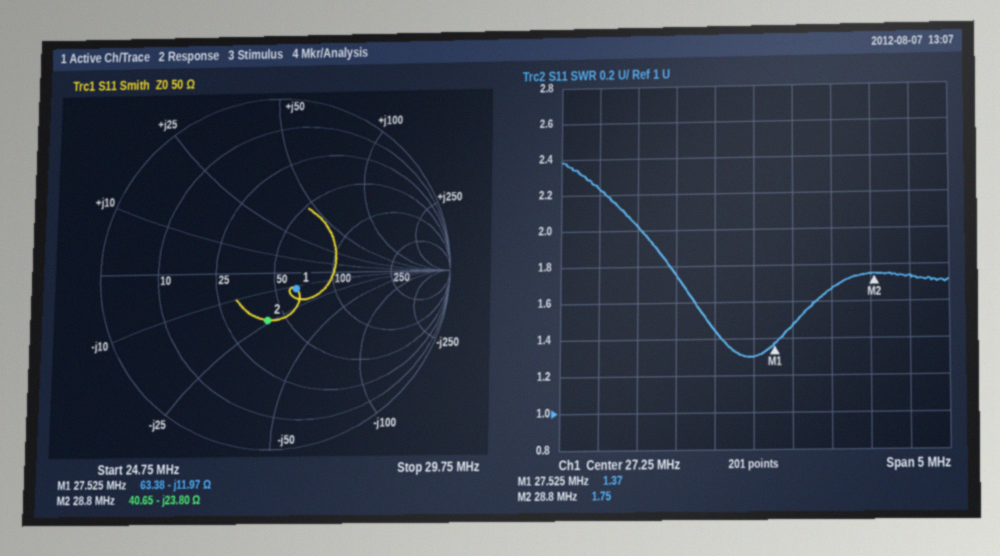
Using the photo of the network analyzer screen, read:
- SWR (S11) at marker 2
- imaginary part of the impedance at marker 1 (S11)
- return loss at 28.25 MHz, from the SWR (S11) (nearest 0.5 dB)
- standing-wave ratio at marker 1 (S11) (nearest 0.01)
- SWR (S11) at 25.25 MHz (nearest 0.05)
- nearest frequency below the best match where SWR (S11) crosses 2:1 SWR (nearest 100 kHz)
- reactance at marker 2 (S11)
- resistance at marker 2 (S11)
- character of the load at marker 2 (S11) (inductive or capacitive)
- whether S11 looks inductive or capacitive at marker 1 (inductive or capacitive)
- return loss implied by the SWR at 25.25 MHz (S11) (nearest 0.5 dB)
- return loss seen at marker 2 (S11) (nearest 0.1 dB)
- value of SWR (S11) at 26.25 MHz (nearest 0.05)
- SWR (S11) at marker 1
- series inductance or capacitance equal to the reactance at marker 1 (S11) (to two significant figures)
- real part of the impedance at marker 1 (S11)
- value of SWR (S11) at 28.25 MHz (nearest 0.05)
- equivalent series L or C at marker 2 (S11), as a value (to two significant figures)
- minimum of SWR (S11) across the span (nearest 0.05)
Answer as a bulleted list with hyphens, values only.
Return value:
- 1.75
- -11.97 Ω
- 12.0 dB
- 1.37
- 2.25
- 25.8 MHz
- -23.80 Ω
- 40.65 Ω
- capacitive
- capacitive
- 8.5 dB
- 11.3 dB
- 1.75
- 1.37
- 480 pF
- 63.38 Ω
- 1.65
- 230 pF
- 1.30
